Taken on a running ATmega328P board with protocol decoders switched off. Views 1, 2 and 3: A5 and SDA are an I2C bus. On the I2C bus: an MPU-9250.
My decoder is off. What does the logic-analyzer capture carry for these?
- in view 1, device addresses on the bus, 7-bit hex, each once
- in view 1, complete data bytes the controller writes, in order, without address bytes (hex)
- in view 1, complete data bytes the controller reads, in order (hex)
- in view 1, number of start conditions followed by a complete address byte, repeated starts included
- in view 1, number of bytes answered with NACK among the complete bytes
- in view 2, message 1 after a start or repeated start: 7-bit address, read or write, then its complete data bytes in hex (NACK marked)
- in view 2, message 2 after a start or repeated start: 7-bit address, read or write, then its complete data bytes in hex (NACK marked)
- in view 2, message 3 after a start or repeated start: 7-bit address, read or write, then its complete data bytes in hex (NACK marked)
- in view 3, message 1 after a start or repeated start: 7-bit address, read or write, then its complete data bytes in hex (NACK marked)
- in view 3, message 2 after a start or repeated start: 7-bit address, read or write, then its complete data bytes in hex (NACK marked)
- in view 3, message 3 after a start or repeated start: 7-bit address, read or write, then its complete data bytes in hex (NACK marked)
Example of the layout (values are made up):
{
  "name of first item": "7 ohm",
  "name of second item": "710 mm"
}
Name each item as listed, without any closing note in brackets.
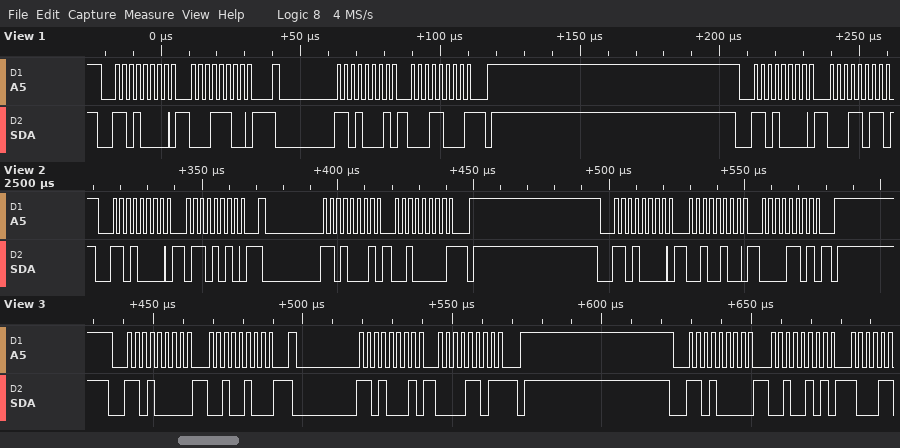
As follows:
{
  "in view 1, device addresses on the bus, 7-bit hex, each once": "0x68",
  "in view 1, complete data bytes the controller writes, in order, without address bytes": "1C 1B",
  "in view 1, complete data bytes the controller reads, in order": "18",
  "in view 1, number of start conditions followed by a complete address byte, repeated starts included": "3",
  "in view 1, number of bytes answered with NACK among the complete bytes": "1",
  "in view 2, message 1 after a start or repeated start: 7-bit address, read or write, then its complete data bytes in hex": "0x68 write: 6A",
  "in view 2, message 2 after a start or repeated start: 7-bit address, read or write, then its complete data bytes in hex": "0x68 read: 20 NACK",
  "in view 2, message 3 after a start or repeated start: 7-bit address, read or write, then its complete data bytes in hex": "0x68 write: 24 0D",
  "in view 3, message 1 after a start or repeated start: 7-bit address, read or write, then its complete data bytes in hex": "0x68 write: 24",
  "in view 3, message 2 after a start or repeated start: 7-bit address, read or write, then its complete data bytes in hex": "0x68 read: 0D NACK",
  "in view 3, message 3 after a start or repeated start: 7-bit address, read or write, then its complete data bytes in hex": "0x68 write: 25"
}
